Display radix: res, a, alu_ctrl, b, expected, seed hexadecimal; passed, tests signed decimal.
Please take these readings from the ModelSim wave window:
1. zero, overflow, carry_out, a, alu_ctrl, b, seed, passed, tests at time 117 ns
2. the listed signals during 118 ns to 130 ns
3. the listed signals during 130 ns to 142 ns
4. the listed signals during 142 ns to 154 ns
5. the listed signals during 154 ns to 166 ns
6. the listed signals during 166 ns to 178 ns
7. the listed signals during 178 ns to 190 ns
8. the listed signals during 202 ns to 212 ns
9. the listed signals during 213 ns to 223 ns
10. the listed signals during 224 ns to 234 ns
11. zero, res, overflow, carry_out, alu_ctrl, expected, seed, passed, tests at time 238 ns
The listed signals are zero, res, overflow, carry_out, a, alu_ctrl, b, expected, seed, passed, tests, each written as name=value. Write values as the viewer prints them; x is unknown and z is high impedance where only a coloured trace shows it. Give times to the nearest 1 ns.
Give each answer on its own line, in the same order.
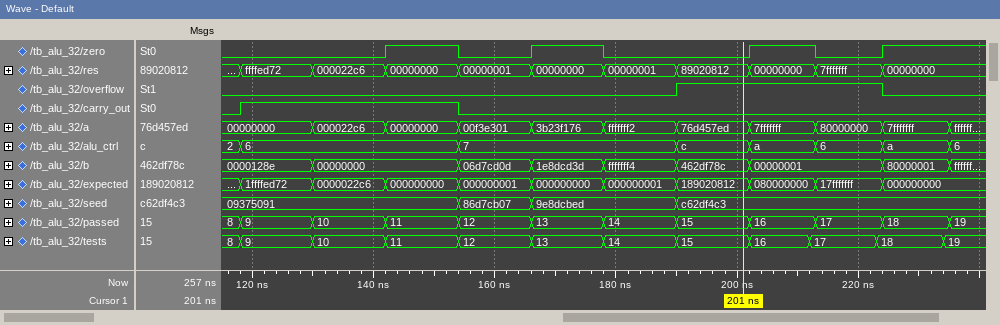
zero=0, overflow=0, carry_out=0, a=00000000, alu_ctrl=2, b=0000128e, seed=09375091, passed=8, tests=8
zero=0, res=ffffed72, overflow=0, carry_out=1, a=00000000, alu_ctrl=6, b=0000128e, expected=1ffffed72, seed=09375091, passed=9, tests=9
zero=0, res=000022c6, overflow=0, carry_out=1, a=000022c6, alu_ctrl=6, b=00000000, expected=0000022c6, seed=09375091, passed=10, tests=10
zero=1, res=00000000, overflow=0, carry_out=1, a=00000000, alu_ctrl=6, b=00000000, expected=000000000, seed=09375091, passed=11, tests=11
zero=0, res=00000001, overflow=0, carry_out=0, a=00f3e301, alu_ctrl=7, b=06d7cd0d, expected=000000001, seed=86d7cb07, passed=12, tests=12
zero=1, res=00000000, overflow=0, carry_out=0, a=3b23f176, alu_ctrl=7, b=1e8dcd3d, expected=000000000, seed=9e8dcbed, passed=13, tests=13
zero=0, res=00000001, overflow=0, carry_out=0, a=fffffff2, alu_ctrl=7, b=fffffff4, expected=000000001, seed=9e8dcbed, passed=14, tests=14
zero=1, res=00000000, overflow=1, carry_out=0, a=7fffffff, alu_ctrl=a, b=00000001, expected=080000000, seed=c62df4c3, passed=16, tests=16
zero=0, res=7fffffff, overflow=1, carry_out=0, a=80000000, alu_ctrl=6, b=00000001, expected=17fffffff, seed=c62df4c3, passed=17, tests=17
zero=1, res=00000000, overflow=0, carry_out=0, a=7fffffff, alu_ctrl=a, b=80000001, expected=000000000, seed=c62df4c3, passed=18, tests=18
zero=1, res=00000000, overflow=0, carry_out=0, alu_ctrl=6, expected=000000000, seed=c62df4c3, passed=19, tests=19
